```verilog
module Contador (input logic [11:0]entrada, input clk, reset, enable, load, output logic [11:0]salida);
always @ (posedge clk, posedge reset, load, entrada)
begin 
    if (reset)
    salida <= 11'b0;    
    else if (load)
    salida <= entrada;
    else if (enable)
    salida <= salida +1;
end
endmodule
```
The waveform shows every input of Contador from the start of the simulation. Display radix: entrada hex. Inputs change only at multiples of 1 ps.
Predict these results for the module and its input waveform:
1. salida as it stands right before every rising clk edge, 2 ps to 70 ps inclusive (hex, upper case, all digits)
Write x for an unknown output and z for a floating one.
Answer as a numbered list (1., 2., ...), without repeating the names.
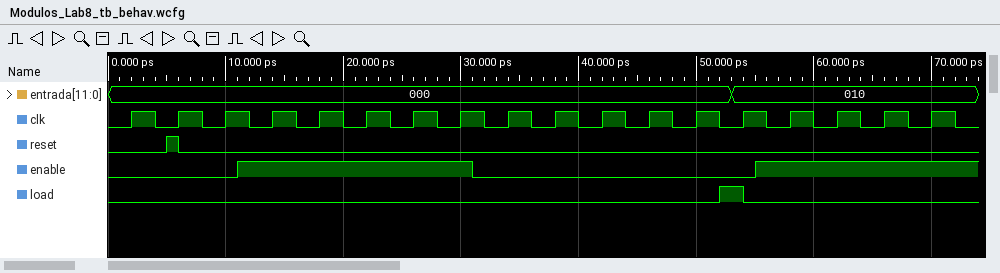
1. x, 000, 000, 000, 001, 002, 003, 004, 005, 005, 005, 005, 005, 010, 010, 011, 012, 013
